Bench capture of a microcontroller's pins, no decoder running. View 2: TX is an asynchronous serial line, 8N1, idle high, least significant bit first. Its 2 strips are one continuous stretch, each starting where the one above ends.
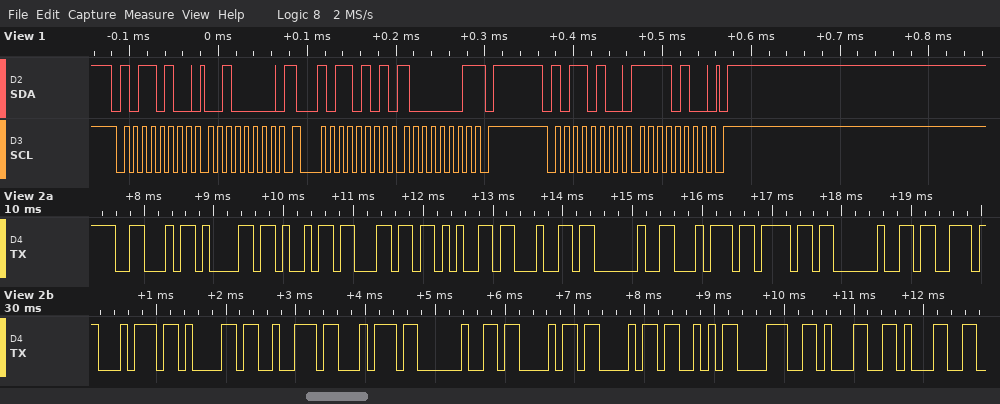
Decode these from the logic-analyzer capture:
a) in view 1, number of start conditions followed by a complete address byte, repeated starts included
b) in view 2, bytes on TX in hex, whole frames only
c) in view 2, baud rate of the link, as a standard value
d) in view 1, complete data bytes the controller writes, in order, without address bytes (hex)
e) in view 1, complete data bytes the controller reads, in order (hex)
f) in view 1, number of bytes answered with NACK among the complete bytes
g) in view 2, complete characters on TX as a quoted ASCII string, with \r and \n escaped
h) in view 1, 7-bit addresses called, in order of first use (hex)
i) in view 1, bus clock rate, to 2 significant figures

3
0x46 0x61 0x69 0x6C 0x65 0x64 0x20 0x74 0x6F 0x20 0x73 0x74 0x61 0x72 0x74 0x20 0x43 0x43 0x53 0x38 0x31 0x31
9600 baud
20 F4
81
1
"Failed to start CCS811"
0x5A
100 kHz
